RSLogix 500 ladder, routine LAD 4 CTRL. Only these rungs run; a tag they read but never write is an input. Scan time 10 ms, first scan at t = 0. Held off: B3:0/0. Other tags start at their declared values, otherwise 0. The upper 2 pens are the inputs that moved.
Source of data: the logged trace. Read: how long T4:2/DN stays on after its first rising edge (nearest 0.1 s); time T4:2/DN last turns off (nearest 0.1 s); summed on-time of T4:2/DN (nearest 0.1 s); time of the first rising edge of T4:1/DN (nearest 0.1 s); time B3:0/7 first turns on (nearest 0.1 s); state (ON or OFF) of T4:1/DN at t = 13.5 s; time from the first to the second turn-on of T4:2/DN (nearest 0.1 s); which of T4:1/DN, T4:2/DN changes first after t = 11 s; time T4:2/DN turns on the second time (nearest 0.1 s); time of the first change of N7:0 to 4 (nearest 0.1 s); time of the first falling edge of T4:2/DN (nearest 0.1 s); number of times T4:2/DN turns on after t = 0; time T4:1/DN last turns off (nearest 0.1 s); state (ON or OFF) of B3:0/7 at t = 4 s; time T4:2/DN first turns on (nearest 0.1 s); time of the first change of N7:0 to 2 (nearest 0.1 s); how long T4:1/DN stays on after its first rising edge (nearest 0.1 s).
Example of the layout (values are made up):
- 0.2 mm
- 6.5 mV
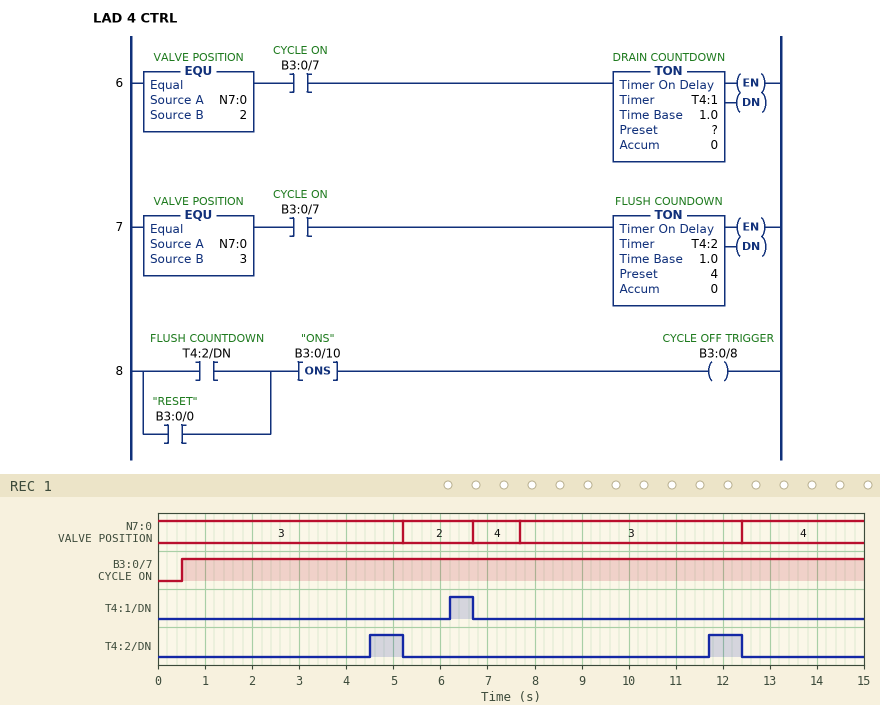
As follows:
- 0.7 s
- 12.4 s
- 1.4 s
- 6.2 s
- 0.5 s
- OFF
- 7.2 s
- T4:2/DN
- 11.7 s
- 6.7 s
- 5.2 s
- 2
- 6.7 s
- ON
- 4.5 s
- 5.2 s
- 0.5 s
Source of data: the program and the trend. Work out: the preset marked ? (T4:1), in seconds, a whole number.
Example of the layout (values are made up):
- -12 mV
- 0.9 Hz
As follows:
- 1 s
